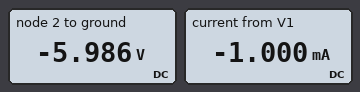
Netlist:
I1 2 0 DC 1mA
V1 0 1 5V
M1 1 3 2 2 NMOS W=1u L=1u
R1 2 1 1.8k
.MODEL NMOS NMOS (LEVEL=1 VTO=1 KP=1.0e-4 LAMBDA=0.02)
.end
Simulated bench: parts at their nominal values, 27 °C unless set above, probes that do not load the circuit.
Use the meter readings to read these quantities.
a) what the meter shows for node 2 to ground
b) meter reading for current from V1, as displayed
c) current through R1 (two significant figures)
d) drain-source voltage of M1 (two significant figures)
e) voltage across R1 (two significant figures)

-5.986 V
-1.000 mA
550 µA
990 mV
990 mV
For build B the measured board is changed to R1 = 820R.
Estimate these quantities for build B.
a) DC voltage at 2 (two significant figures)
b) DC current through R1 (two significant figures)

-5.6 V
740 µA
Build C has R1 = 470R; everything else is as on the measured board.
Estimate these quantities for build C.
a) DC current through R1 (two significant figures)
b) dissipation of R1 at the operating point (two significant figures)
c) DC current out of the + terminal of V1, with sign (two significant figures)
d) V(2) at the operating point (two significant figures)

830 µA
330 µW
-1.0 mA
-5.4 V
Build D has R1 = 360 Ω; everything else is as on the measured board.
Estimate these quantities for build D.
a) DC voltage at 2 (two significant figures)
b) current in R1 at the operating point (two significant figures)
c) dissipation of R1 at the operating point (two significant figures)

-5.3 V
870 µA
270 µW
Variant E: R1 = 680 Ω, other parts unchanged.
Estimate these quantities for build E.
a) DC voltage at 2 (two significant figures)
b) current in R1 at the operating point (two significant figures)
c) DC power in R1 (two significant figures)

-5.5 V
770 µA
410 µW
